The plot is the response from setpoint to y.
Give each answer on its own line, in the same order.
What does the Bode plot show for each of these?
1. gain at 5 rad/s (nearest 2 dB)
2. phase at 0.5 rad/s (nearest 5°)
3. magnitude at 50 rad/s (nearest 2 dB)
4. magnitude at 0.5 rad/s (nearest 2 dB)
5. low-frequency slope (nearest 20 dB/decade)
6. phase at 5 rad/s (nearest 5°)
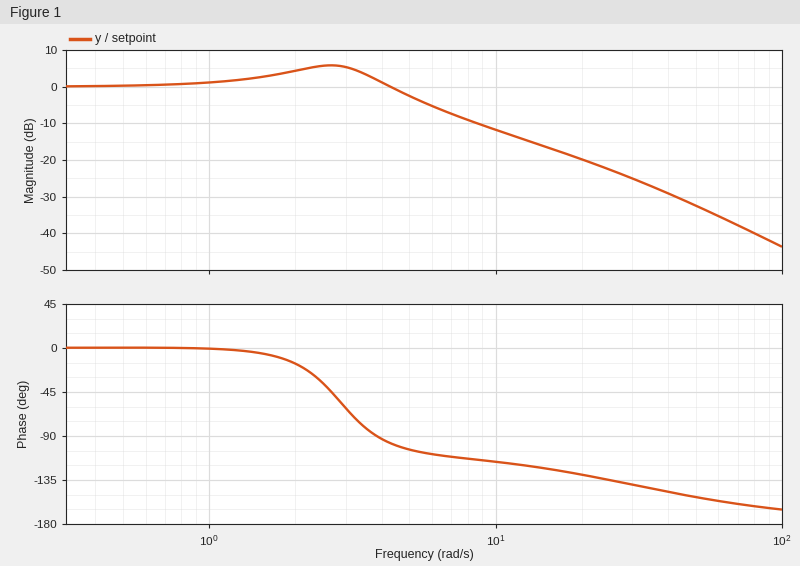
-2 dB
0°
-32 dB
0 dB
0 dB/decade
-105°
